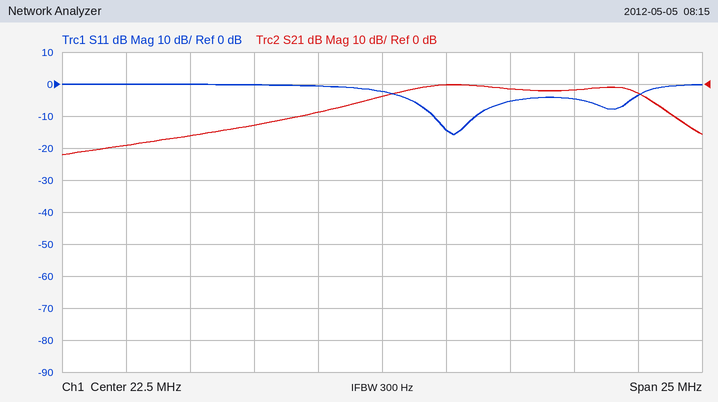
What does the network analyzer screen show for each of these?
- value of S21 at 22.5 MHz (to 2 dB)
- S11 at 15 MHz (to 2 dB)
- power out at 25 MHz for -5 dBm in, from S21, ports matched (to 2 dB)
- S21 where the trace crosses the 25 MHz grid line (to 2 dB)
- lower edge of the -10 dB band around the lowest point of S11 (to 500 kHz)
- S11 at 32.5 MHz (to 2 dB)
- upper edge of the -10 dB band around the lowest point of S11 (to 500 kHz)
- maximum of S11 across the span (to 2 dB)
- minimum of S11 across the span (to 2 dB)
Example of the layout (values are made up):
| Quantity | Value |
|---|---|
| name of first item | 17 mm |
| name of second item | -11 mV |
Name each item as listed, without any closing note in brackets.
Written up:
| Quantity | Value |
|---|---|
| value of S21 at 22.5 MHz | -4 dB |
| S11 at 15 MHz | 0 dB |
| power out at 25 MHz for -5 dBm in, from S21, ports matched | -6 dBm |
| S21 where the trace crosses the 25 MHz grid line | 0 dB |
| lower edge of the -10 dB band around the lowest point of S11 | 24.5 MHz |
| S11 at 32.5 MHz | -4 dB |
| upper edge of the -10 dB band around the lowest point of S11 | 26.0 MHz |
| maximum of S11 across the span | 0 dB |
| minimum of S11 across the span | -16 dB |
